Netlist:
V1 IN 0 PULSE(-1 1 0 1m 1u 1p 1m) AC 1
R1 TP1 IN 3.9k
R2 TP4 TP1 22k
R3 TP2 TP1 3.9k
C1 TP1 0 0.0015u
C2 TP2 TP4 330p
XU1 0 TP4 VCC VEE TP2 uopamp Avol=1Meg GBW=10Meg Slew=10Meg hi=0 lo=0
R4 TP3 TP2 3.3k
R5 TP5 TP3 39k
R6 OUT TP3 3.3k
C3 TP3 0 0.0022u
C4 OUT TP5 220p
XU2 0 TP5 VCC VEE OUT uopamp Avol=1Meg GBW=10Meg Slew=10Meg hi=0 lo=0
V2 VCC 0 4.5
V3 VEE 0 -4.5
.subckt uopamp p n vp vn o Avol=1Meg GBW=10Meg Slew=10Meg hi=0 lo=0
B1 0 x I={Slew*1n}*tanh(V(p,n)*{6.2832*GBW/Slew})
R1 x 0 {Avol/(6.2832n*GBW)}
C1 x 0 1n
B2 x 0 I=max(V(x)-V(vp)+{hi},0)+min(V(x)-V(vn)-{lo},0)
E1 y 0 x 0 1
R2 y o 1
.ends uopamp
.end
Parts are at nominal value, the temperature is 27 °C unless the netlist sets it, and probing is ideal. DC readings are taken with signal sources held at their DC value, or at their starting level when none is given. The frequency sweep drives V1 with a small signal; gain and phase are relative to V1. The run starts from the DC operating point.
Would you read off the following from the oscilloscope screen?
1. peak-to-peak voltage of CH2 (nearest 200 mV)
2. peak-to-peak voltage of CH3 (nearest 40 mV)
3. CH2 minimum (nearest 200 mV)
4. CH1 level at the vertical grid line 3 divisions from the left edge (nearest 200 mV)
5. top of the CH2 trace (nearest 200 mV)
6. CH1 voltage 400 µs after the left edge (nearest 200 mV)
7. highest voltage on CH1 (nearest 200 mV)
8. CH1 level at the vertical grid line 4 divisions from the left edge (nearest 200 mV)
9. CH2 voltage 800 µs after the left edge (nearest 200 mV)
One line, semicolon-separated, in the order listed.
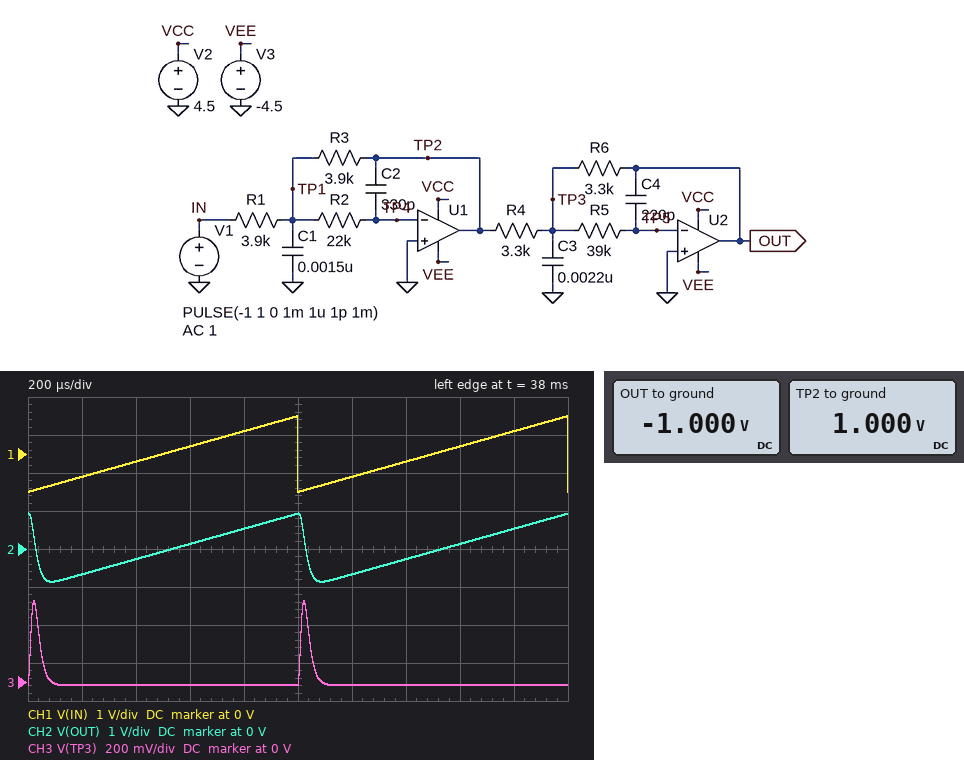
1.8 V; 440 mV; -800 mV; 200 mV; 1.0 V; -200 mV; 1.0 V; 600 mV; 600 mV
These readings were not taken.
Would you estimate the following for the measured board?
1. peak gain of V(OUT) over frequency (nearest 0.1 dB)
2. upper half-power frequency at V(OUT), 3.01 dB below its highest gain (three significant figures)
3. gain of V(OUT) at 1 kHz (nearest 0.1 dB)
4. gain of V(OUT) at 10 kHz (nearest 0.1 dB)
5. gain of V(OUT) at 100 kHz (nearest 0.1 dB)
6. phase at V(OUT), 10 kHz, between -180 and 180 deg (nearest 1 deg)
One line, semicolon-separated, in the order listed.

0 dB; 7.50 kHz; -0.1 dB; -4.9 dB; -53.8 dB; -106 deg
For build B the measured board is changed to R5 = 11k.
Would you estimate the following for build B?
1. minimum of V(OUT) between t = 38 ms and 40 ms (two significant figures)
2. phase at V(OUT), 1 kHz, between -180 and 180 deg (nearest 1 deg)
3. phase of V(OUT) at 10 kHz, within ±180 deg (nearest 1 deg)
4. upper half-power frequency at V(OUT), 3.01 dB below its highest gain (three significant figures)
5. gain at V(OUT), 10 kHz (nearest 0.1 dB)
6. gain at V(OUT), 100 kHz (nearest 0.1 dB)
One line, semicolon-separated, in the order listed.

-890 mV; -8 deg; -71 deg; 12.2 kHz; -2.2 dB; -42.2 dB
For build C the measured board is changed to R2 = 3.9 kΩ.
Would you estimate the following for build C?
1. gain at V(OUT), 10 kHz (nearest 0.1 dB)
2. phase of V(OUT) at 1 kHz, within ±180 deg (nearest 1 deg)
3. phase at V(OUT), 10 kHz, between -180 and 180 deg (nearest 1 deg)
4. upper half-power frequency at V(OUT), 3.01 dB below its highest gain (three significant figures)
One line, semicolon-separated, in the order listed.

-2.6 dB; -8 deg; -70 deg; 10.9 kHz
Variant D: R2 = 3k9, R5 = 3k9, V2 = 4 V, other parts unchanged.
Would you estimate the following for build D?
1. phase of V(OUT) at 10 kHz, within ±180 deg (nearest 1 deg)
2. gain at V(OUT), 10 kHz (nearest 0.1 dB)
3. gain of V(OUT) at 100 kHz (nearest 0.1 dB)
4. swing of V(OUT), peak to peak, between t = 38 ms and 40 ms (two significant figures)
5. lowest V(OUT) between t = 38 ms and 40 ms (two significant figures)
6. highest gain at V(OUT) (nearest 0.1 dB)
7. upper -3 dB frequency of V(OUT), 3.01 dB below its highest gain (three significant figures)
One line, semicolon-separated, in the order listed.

-23 deg; 0.1 dB; -16.7 dB; 2.3 V; -1.3 V; 0.6 dB; 58.8 kHz
